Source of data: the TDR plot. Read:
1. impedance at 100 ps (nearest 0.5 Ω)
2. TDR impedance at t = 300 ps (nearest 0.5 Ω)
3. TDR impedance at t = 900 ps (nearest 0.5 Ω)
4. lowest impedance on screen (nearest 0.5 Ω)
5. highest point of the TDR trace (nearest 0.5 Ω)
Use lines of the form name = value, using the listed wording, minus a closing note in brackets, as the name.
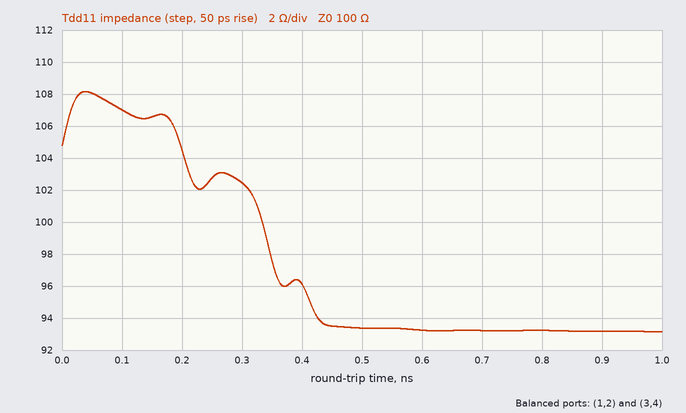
impedance at 100 ps = 107.0 Ω
TDR impedance at t = 300 ps = 102.5 Ω
TDR impedance at t = 900 ps = 93.0 Ω
lowest impedance on screen = 93.0 Ω
highest point of the TDR trace = 108.0 Ω
